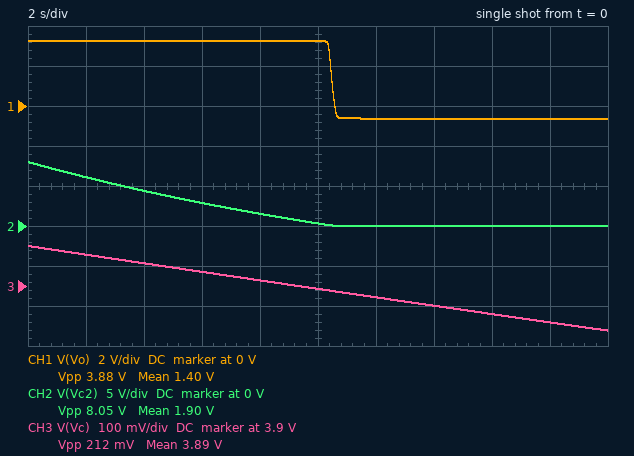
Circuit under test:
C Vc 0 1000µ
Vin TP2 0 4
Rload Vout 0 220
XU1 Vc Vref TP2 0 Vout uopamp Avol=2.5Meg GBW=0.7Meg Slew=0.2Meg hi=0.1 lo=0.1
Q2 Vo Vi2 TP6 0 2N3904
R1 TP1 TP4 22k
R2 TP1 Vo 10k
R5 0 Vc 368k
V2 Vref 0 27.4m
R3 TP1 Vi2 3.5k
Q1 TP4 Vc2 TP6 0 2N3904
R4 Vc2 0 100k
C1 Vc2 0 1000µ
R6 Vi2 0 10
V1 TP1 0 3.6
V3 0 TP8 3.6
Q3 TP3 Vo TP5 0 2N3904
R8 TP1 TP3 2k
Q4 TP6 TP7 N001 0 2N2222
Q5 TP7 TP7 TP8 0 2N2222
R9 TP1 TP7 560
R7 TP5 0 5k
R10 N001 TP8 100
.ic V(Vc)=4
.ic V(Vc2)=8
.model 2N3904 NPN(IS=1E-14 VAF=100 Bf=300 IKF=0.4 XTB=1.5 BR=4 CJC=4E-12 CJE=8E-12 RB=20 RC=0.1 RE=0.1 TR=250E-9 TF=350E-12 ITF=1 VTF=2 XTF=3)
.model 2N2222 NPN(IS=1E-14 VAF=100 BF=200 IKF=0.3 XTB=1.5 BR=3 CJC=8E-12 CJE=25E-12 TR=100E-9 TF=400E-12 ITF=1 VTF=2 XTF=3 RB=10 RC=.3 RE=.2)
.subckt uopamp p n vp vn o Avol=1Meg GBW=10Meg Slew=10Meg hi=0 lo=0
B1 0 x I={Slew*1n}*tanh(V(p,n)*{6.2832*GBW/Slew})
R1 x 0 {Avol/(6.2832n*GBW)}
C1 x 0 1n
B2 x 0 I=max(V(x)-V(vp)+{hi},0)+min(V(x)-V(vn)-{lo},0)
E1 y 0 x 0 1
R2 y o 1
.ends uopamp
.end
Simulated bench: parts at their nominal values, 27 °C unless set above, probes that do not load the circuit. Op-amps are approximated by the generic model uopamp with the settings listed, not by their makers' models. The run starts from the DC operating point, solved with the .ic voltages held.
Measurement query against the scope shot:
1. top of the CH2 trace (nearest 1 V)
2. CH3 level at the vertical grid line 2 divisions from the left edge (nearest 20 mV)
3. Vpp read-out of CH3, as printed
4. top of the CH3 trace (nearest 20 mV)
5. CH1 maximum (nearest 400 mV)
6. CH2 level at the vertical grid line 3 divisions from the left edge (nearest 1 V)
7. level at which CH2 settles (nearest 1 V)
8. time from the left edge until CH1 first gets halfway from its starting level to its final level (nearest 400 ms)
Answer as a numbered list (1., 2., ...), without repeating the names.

1. 8 V
2. 3.96 V
3. 212 mV
4. 4.00 V
5. 3.2 V
6. 3 V
7. 0 V
8. 10.4 s
